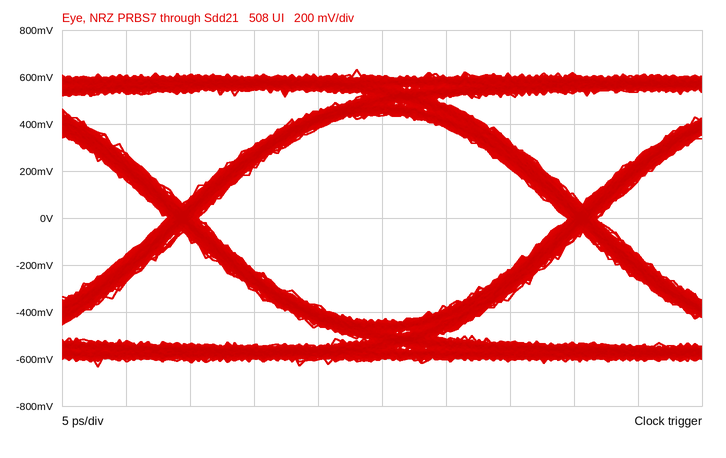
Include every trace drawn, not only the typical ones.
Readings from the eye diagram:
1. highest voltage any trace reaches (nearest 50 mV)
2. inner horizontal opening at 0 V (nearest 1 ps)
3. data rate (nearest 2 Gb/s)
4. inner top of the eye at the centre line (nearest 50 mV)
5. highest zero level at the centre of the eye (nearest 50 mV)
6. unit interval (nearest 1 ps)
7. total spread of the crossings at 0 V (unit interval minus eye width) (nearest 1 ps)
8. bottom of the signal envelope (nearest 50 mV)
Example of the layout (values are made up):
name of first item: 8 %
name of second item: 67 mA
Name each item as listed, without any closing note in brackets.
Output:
highest voltage any trace reaches: 650 mV
inner horizontal opening at 0 V: 29 ps
data rate: 32 Gb/s
inner top of the eye at the centre line: 450 mV
highest zero level at the centre of the eye: -450 mV
unit interval: 31 ps
total spread of the crossings at 0 V (unit interval minus eye width): 2 ps
bottom of the signal envelope: -650 mV
